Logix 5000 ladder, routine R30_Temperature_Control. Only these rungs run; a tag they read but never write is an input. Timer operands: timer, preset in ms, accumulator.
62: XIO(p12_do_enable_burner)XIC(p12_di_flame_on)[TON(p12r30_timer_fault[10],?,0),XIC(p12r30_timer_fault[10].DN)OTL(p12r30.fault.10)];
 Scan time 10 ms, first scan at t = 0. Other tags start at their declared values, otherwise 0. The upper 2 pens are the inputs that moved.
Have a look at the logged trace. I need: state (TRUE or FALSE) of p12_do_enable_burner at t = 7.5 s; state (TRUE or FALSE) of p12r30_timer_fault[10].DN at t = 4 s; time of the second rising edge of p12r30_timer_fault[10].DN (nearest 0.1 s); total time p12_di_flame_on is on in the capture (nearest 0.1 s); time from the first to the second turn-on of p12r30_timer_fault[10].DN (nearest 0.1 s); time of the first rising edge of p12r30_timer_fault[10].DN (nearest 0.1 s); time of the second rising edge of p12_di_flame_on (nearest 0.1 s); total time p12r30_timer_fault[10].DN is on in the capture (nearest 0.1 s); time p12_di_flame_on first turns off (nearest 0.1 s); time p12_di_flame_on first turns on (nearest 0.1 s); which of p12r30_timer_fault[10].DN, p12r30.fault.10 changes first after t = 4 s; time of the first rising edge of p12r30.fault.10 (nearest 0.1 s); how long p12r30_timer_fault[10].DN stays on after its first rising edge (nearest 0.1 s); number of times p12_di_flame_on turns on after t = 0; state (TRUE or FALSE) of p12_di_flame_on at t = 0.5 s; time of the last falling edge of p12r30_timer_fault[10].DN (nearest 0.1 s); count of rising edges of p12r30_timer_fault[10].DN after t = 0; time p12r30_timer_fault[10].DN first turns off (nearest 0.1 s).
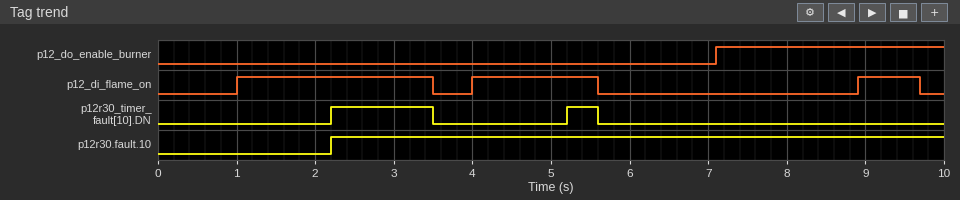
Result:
TRUE
FALSE
5.2 s
4.9 s
3.0 s
2.2 s
4.0 s
1.7 s
3.5 s
1.0 s
p12r30_timer_fault[10].DN
2.2 s
1.3 s
3
FALSE
5.6 s
2
3.5 s
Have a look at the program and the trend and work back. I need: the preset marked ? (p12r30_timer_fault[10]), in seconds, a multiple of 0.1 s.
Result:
1.2 s
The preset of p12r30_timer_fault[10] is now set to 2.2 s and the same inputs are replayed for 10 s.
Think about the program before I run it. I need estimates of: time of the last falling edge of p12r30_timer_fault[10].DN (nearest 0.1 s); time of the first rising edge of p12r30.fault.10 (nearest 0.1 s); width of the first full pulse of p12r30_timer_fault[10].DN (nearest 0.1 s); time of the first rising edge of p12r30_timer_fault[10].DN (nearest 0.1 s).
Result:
3.5 s
3.2 s
0.3 s
3.2 s
